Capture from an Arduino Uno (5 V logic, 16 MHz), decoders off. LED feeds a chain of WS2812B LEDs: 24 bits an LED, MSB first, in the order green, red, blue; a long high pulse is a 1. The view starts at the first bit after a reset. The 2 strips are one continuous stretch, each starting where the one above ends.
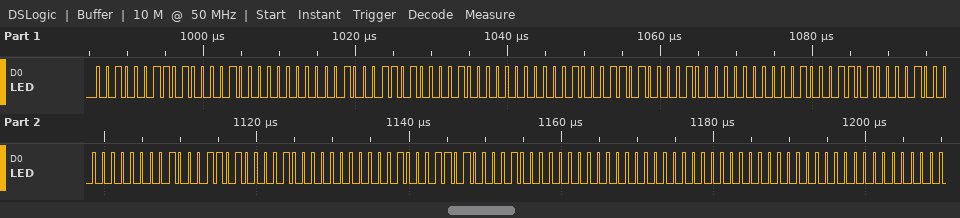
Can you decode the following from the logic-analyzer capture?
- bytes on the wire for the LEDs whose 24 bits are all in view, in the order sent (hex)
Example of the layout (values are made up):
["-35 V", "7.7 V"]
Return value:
["23 42 00 23 42 00 23 42 00 23 42 00 23 42 00 23 42 00 00 00 00"]
